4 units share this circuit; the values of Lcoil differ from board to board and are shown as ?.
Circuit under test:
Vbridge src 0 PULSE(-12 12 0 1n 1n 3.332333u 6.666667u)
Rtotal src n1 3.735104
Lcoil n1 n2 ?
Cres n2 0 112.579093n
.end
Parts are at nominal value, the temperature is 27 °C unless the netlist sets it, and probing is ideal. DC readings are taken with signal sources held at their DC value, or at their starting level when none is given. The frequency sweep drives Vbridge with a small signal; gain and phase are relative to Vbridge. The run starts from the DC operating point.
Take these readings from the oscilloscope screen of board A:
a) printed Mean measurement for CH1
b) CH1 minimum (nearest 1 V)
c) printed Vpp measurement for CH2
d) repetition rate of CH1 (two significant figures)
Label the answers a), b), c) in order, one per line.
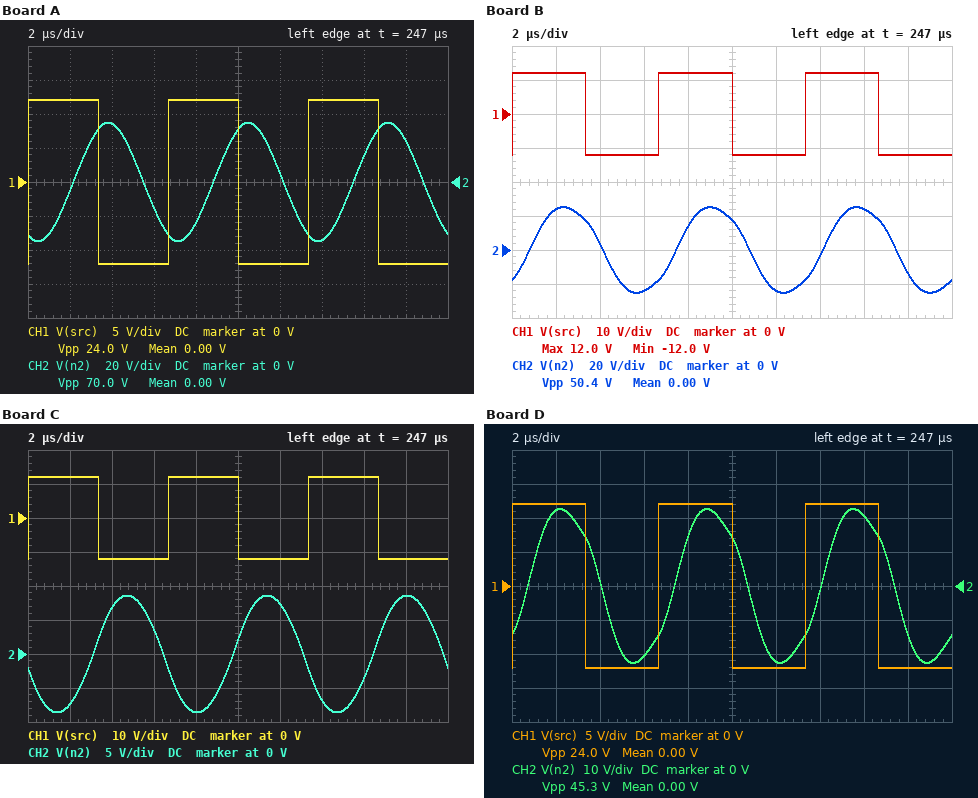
a) 0.00 V
b) -12 V
c) 70.0 V
d) 150 kHz
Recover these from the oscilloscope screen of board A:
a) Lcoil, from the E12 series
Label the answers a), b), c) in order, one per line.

a) 12 µH
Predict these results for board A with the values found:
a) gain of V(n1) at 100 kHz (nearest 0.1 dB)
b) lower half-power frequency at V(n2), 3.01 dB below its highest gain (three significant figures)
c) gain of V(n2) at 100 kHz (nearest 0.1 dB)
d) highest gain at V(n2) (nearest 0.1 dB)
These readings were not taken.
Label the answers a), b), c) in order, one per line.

a) -1.2 dB
b) 104 kHz
c) 5.4 dB
d) 9.0 dB
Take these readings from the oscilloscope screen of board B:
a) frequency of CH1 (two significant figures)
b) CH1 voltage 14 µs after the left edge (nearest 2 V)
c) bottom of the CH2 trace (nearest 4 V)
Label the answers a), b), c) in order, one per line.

a) 150 kHz
b) 12 V
c) -24 V
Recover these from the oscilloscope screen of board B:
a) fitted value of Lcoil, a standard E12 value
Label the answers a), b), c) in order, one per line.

a) 5.6 µH
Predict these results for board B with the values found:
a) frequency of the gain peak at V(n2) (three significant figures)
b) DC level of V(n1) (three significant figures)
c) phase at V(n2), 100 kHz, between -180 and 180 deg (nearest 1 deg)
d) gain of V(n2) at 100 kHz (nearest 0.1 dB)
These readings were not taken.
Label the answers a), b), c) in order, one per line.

a) 186 kHz
b) -12.0 V
c) -19 deg
d) 2.0 dB
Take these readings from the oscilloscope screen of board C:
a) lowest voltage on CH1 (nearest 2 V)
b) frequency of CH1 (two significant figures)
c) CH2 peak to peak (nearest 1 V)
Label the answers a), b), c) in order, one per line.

a) -12 V
b) 150 kHz
c) 17 V
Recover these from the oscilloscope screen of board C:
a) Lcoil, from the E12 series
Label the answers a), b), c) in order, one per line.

a) 27 µH
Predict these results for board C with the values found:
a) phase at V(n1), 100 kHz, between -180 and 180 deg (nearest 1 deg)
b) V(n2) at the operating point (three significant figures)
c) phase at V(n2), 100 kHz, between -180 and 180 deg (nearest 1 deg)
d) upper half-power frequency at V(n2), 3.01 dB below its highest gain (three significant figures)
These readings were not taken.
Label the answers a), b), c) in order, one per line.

a) 53 deg
b) -12.0 V
c) -127 deg
d) 100 kHz
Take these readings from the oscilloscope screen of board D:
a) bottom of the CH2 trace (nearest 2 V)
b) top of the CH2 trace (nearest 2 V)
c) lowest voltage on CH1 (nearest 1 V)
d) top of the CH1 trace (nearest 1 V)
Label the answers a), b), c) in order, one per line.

a) -22 V
b) 22 V
c) -12 V
d) 12 V
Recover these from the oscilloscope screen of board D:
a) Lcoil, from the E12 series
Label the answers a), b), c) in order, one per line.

a) 4.7 µH
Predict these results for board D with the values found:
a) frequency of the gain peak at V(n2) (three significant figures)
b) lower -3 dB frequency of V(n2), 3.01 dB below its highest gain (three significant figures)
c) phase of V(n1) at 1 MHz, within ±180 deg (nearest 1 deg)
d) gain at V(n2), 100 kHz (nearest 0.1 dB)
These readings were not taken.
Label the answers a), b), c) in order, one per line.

a) 200 kHz
b) 116 kHz
c) 8 deg
d) 1.6 dB
